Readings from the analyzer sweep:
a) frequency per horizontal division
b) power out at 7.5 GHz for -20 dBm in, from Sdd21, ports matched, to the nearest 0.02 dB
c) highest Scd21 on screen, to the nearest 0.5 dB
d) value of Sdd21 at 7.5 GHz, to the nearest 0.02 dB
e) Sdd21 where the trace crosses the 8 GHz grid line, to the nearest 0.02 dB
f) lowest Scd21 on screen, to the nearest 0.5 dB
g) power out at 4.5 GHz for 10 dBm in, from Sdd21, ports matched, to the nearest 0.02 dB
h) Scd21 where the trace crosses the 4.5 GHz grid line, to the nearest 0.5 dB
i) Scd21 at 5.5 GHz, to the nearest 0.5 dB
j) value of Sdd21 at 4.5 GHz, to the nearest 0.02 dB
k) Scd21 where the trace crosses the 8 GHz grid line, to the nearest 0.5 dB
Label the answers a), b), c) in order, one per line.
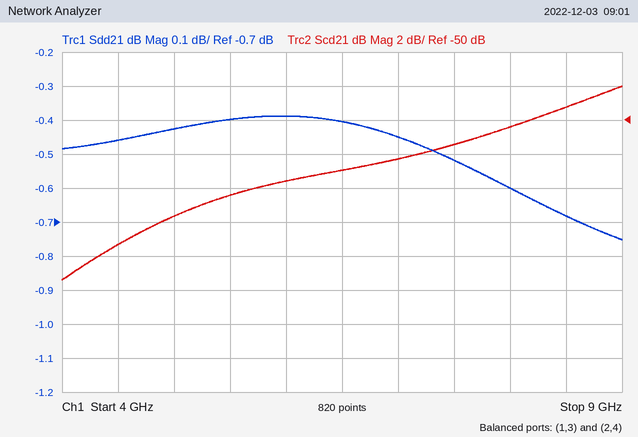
a) 500 MHz
b) -20.52 dBm
c) -48.0 dB
d) -0.52 dB
e) -0.60 dB
f) -59.5 dB
g) 9.54 dBm
h) -57.5 dB
i) -54.5 dB
j) -0.46 dB
k) -50.5 dB
